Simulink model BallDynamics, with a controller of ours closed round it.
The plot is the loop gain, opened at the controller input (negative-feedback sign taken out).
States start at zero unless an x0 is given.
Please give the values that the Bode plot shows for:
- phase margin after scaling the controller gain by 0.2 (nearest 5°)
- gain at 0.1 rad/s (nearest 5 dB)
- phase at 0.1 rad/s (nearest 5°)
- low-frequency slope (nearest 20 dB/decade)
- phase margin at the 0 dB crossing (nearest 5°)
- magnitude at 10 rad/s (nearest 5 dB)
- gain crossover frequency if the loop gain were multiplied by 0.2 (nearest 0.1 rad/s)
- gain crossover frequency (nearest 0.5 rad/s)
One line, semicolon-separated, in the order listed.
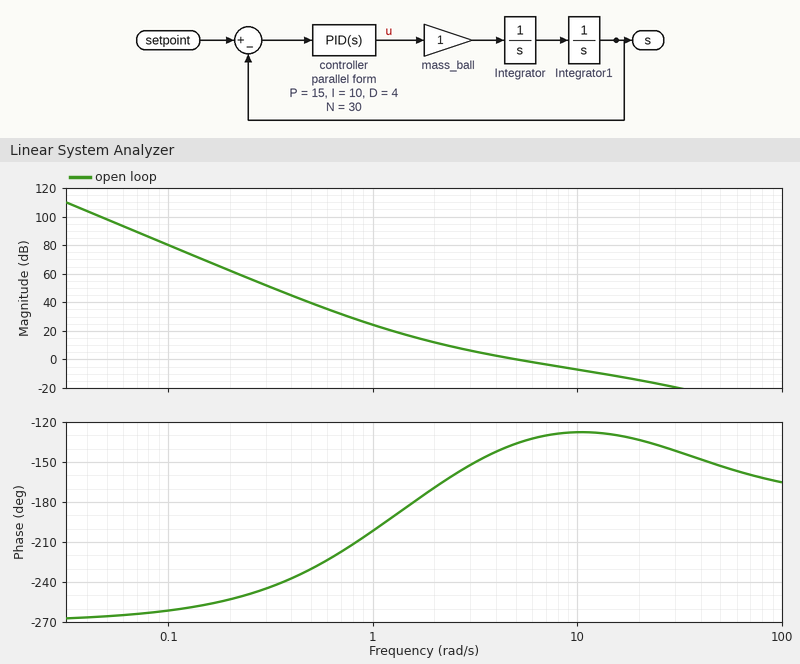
5°; 80 dB; -260°; -60 dB/decade; 45°; -5 dB; 1.8 rad/s; 5.0 rad/s
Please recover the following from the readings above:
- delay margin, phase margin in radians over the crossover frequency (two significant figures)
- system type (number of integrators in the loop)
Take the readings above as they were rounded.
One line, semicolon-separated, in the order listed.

0.16 s; 3
